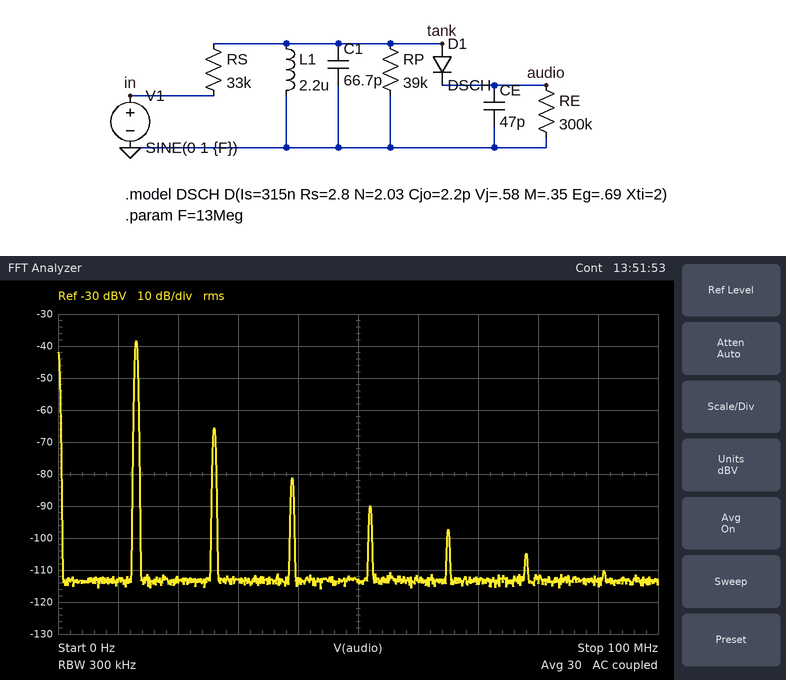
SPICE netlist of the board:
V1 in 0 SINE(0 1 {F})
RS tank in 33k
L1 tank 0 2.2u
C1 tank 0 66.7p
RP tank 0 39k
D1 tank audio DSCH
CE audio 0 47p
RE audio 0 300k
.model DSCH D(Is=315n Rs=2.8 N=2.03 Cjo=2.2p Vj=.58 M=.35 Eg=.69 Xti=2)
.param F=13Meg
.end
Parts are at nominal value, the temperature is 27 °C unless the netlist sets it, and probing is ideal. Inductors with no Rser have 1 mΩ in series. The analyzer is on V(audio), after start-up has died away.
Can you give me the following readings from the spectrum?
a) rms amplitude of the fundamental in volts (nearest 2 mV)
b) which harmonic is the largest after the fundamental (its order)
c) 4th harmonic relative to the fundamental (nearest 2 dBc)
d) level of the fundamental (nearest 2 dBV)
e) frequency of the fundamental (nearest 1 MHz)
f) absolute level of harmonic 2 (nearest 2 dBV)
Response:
12 mV
2
-52 dBc
-38 dBV
13 MHz
-66 dBV
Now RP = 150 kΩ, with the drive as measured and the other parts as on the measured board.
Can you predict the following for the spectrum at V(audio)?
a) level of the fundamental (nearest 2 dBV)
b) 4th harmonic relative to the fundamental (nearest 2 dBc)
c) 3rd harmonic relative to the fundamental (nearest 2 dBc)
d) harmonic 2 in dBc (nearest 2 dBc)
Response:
-36 dBV
-48 dBc
-40 dBc
-26 dBc
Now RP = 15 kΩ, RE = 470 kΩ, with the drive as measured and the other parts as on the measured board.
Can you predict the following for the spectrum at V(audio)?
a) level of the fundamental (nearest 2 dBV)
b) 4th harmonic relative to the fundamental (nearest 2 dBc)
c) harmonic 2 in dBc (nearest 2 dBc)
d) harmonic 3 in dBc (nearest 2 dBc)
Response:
-42 dBV
-58 dBc
-30 dBc
-48 dBc
